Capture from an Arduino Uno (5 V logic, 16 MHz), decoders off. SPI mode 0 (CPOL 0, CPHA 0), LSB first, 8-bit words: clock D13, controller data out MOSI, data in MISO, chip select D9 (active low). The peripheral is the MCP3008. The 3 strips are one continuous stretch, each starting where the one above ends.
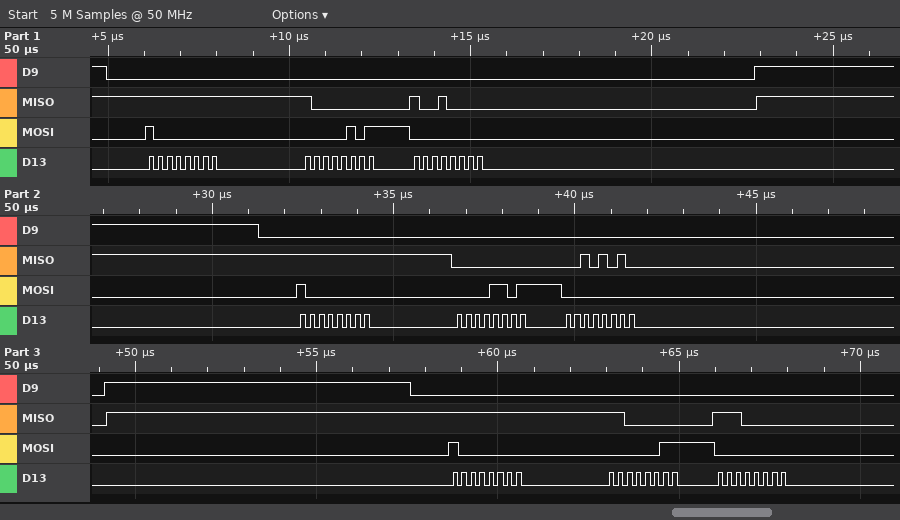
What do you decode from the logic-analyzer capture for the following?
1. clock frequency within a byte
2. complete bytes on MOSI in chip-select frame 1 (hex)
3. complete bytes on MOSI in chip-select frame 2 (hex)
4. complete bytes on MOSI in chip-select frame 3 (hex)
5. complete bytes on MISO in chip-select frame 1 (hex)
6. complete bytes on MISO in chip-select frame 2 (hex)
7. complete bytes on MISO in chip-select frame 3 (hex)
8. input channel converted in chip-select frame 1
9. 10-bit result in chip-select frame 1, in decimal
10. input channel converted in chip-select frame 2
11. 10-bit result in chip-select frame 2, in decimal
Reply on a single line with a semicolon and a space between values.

4 MHz; 01 A0 00; 01 B0 00; 01 C0 00; FF 01 09; FF 00 54; FF 03 07; 2; 265; 3; 84
